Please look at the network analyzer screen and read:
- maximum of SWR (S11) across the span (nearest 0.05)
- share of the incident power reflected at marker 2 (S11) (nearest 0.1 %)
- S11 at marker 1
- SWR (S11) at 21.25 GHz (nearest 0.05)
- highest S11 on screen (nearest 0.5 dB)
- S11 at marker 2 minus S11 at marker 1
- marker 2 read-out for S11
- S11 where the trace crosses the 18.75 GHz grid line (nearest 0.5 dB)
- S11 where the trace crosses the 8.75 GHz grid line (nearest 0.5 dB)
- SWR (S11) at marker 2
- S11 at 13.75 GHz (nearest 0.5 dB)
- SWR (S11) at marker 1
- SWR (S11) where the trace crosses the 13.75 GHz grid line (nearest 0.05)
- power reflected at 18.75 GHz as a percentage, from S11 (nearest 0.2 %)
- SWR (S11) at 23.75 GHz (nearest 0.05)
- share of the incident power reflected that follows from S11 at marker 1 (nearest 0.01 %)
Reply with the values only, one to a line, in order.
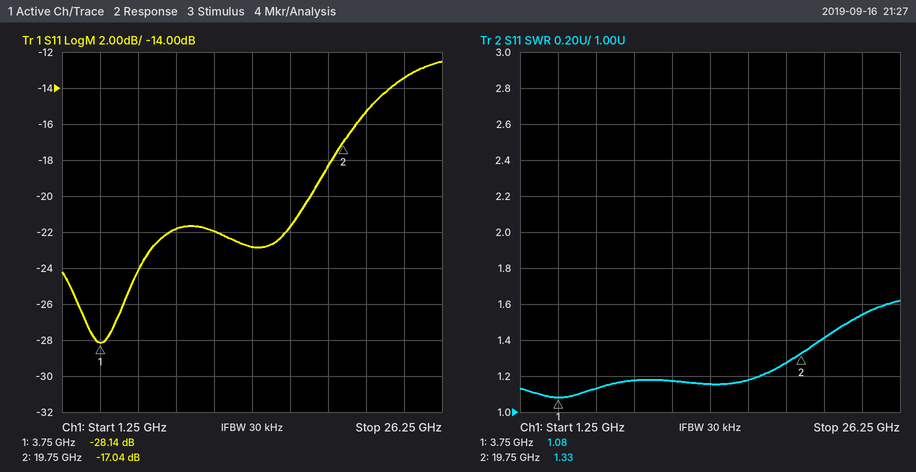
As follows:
1.60
2.0 %
-28.14 dB
1.40
-12.5 dB
11.10 dB
-17.04 dB
-18.5 dB
-22.0 dB
1.33
-23.0 dB
1.08
1.15
1.4 %
1.55
0.15 %
